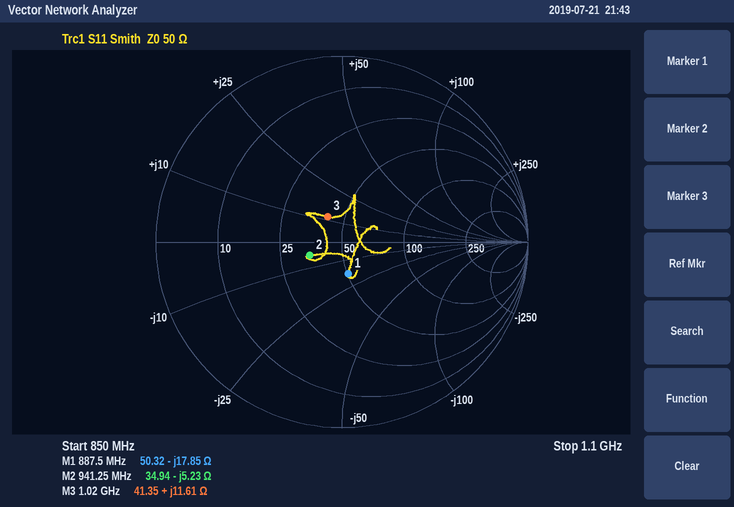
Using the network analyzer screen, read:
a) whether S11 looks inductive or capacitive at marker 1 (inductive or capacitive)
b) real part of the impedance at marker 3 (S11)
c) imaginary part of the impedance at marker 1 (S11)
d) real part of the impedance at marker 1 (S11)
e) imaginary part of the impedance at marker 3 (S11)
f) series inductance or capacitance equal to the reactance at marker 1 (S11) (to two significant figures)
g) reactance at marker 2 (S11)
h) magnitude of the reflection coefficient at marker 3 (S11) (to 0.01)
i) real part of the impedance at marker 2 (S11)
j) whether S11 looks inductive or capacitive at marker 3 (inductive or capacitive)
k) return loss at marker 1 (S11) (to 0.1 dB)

capacitive
41.35 Ω
-17.85 Ω
50.32 Ω
+11.61 Ω
10 pF
-5.23 Ω
0.16
34.94 Ω
inductive
15.1 dB
